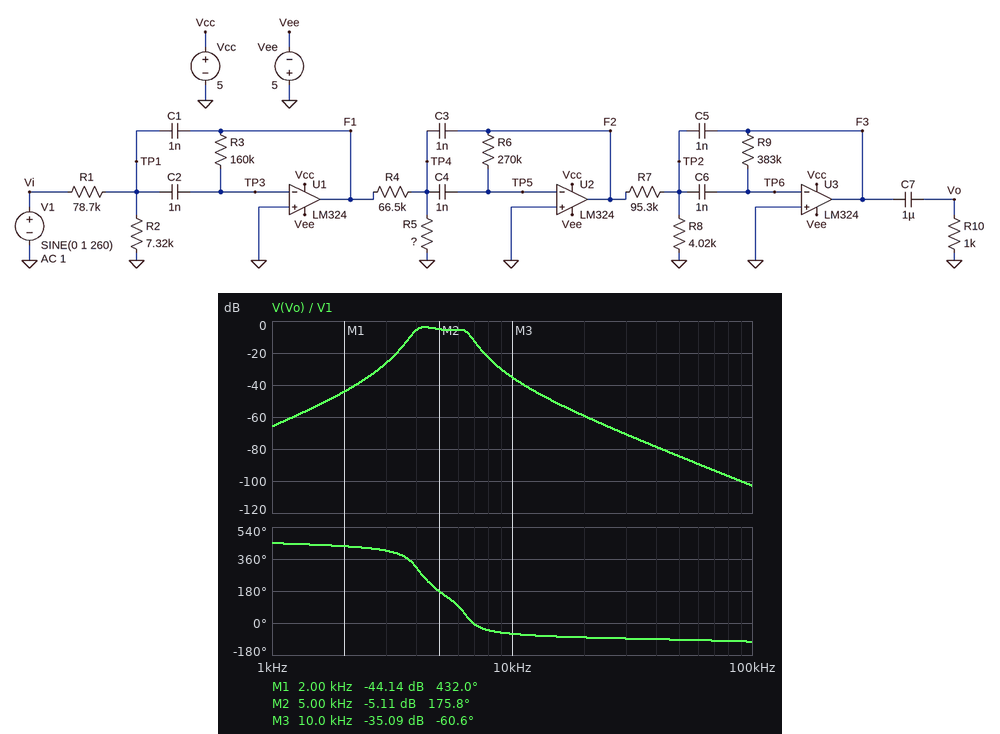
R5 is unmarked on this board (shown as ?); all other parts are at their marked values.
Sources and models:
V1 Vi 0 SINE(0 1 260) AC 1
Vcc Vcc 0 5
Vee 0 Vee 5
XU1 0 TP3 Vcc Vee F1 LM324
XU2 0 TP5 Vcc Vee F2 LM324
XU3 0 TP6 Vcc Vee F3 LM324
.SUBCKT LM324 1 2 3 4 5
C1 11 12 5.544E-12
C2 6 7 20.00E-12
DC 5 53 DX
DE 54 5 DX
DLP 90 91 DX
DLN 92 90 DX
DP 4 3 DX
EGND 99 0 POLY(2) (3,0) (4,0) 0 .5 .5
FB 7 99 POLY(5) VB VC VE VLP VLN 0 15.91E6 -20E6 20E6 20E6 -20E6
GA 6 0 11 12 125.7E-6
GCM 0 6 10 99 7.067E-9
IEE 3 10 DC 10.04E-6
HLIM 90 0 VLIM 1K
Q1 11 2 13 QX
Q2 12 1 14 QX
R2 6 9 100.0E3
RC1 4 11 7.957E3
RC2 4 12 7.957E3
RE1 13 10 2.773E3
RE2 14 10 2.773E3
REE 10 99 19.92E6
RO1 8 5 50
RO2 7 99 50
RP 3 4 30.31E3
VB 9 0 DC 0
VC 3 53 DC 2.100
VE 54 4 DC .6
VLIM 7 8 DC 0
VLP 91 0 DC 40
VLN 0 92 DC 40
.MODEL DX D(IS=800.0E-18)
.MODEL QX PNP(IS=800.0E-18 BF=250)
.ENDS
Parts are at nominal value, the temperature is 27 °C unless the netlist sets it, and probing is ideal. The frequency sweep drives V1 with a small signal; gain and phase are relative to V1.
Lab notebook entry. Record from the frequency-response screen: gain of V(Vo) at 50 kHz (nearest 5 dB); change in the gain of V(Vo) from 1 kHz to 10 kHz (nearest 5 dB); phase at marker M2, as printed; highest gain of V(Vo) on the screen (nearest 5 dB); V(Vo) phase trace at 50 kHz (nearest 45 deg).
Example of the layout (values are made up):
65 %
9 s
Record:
-85 dB
30 dB
175.8 deg
-5 dB
-90 deg
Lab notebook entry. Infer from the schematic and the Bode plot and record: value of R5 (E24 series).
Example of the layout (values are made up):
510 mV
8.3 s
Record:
2.2 kΩ
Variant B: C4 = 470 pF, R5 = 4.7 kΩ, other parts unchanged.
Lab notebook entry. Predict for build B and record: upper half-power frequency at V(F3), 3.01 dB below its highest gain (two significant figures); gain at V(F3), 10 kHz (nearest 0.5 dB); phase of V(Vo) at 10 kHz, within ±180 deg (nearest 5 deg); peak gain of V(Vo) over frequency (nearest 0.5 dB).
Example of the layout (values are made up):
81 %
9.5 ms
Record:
5.4 kHz
-34.5 dB
-55 deg
-5.0 dB
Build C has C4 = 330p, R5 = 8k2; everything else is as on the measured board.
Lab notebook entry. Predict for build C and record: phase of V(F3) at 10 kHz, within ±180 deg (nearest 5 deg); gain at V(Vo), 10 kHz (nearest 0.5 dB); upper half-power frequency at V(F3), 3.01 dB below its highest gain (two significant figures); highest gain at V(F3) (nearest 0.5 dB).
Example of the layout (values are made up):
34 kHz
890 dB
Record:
-50 deg
-35.5 dB
5.3 kHz
-3.0 dB
